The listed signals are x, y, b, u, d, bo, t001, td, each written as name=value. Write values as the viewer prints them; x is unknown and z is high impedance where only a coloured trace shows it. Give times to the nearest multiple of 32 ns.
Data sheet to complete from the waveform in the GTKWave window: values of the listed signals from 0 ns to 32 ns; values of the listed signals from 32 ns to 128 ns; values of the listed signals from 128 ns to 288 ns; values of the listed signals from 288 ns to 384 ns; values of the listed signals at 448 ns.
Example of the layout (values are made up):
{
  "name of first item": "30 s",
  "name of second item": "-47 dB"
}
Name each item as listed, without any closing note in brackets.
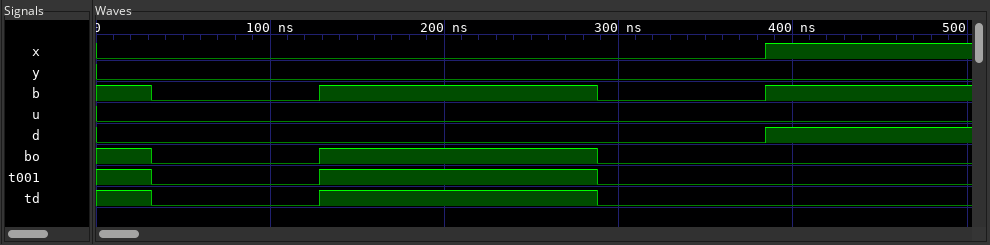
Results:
{
  "values of the listed signals from 0 ns to 32 ns": "x=0, y=0, b=1, u=0, d=0, bo=1, t001=1, td=1",
  "values of the listed signals from 32 ns to 128 ns": "x=0, y=0, b=0, u=0, d=0, bo=0, t001=0, td=0",
  "values of the listed signals from 128 ns to 288 ns": "x=0, y=0, b=1, u=0, d=0, bo=1, t001=1, td=1",
  "values of the listed signals from 288 ns to 384 ns": "x=0, y=0, b=0, u=0, d=0, bo=0, t001=0, td=0",
  "values of the listed signals at 448 ns": "x=1, y=0, b=1, u=0, d=1, bo=0, t001=0, td=0"
}
